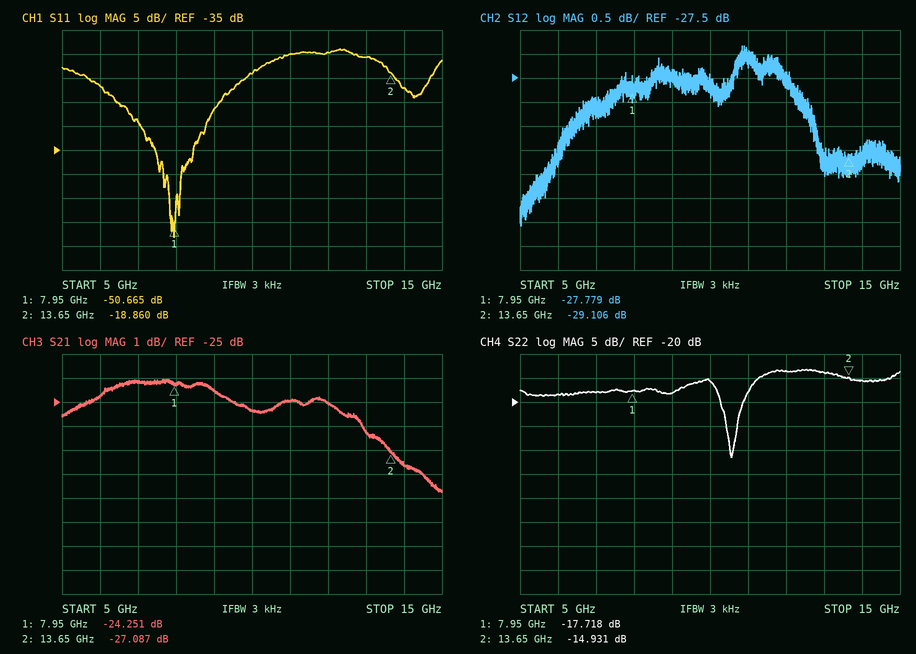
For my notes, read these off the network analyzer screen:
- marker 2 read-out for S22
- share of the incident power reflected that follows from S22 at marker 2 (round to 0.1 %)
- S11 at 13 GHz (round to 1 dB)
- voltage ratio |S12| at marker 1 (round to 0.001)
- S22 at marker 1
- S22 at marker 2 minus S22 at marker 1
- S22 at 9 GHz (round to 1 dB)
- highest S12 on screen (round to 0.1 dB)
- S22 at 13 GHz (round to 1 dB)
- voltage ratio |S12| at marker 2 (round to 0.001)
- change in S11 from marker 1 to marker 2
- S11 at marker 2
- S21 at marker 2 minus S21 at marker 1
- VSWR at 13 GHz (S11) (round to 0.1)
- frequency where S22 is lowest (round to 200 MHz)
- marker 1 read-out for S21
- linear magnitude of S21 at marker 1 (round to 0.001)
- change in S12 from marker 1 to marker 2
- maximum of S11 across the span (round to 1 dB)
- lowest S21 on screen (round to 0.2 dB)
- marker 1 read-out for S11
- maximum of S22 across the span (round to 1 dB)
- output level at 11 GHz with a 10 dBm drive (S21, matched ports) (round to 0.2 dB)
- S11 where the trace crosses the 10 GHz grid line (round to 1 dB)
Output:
-14.931 dB
3.2 %
-16 dB
0.041
-17.718 dB
2.787 dB
-18 dB
-26.8 dB
-14 dB
0.035
31.805 dB
-18.860 dB
-2.836 dB
1.4
10.6 GHz
-24.251 dB
0.061
-1.327 dB
-14 dB
-28.8 dB
-50.665 dB
-13 dB
-15.0 dBm
-19 dB
